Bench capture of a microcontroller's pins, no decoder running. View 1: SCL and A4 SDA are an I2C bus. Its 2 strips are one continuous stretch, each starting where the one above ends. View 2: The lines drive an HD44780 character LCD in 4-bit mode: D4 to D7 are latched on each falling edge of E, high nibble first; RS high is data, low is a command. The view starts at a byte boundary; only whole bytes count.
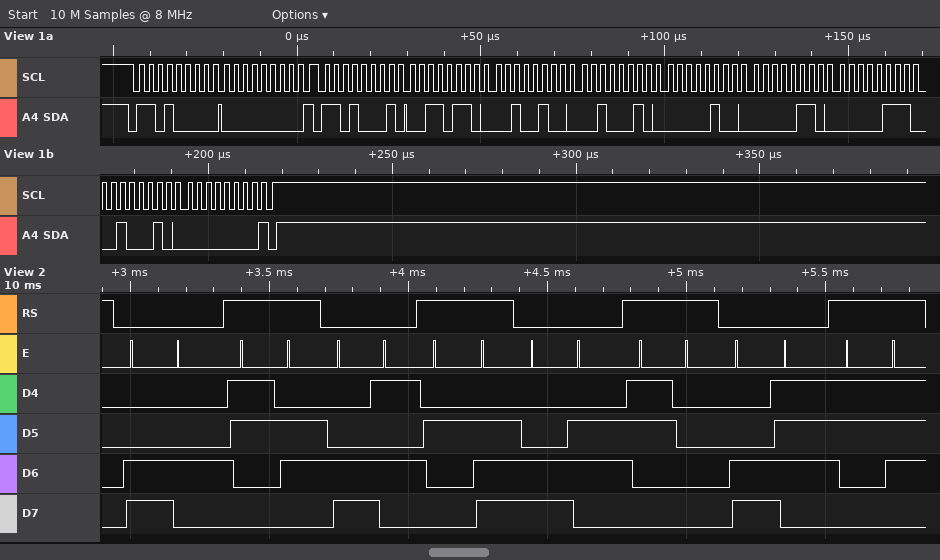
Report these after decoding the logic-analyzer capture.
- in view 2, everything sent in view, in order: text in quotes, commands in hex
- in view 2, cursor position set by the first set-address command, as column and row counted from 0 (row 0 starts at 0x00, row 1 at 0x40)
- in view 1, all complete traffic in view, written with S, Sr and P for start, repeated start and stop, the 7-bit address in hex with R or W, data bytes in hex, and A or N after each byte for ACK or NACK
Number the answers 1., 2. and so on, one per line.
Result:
1. 0xC4 "6" 0xC5 "." 0xC6 "0" 0xC7 "7"
2. column 4, row 1
3. S 68W A 00 A Sr 68R A 36 A 24 A 22 A 04 A 06 A 07 A 22 A 00 N P
